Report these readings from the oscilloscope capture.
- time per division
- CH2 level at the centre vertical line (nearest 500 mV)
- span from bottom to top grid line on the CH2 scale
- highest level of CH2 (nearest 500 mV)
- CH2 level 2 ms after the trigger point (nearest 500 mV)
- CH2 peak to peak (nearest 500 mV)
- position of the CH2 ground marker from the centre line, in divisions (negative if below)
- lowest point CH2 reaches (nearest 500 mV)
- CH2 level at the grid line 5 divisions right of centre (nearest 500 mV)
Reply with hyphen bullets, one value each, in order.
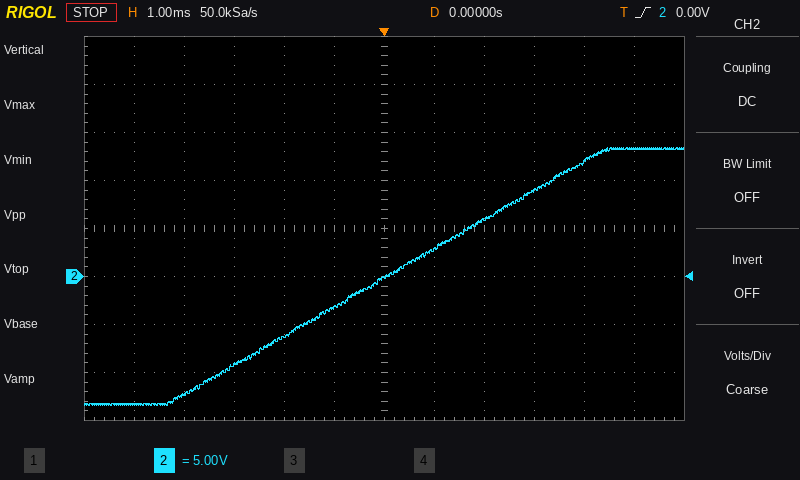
- 1 ms
- 0.0 V
- 40 V
- 13.5 V
- 6.0 V
- 27.0 V
- -1.0 div
- -13.5 V
- 13.5 V
